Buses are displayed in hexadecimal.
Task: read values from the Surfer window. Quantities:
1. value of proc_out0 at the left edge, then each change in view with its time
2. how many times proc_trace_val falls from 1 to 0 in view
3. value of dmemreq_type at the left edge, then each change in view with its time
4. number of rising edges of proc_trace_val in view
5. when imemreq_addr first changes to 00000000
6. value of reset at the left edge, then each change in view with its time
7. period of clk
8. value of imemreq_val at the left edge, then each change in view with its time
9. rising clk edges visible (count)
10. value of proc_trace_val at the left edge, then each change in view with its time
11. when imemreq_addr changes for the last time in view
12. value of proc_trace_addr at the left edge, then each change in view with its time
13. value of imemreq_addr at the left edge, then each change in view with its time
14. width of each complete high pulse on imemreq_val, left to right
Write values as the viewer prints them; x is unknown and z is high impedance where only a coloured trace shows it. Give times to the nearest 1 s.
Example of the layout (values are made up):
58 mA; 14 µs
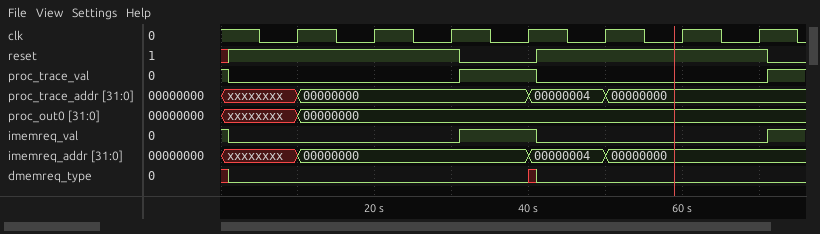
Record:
xxxxxxxx, 00000000 at 10 s; 2; x, 0 at 1 s, x at 40 s, 0 at 41 s; 2; 10 s; x, 1 at 1 s, 0 at 31 s, 1 at 41 s, 0 at 71 s; 10 s; 1, 0 at 1 s, 1 at 31 s, 0 at 41 s, 1 at 71 s; 7; 1, 0 at 1 s, 1 at 31 s, 0 at 41 s, 1 at 71 s; 50 s; xxxxxxxx, 00000000 at 10 s, 00000004 at 40 s, 00000000 at 50 s; xxxxxxxx, 00000000 at 10 s, 00000004 at 40 s, 00000000 at 50 s; 10 s
